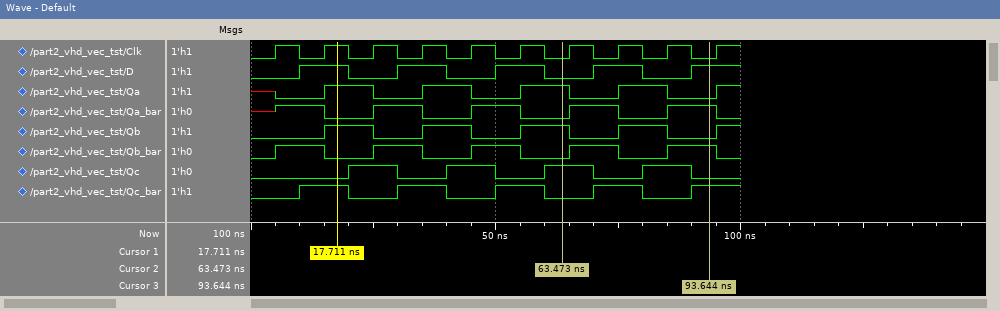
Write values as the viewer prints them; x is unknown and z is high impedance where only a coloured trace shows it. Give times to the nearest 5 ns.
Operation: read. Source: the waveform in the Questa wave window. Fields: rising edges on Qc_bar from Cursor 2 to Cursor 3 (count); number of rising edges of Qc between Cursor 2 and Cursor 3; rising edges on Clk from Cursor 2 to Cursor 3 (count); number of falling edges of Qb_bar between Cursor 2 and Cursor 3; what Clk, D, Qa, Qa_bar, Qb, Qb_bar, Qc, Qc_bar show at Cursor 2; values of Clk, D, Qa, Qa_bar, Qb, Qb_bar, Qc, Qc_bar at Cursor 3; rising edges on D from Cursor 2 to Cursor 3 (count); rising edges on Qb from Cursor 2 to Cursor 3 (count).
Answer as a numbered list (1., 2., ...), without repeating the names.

1. 2
2. 1
3. 3
4. 1
5. Clk=0, D=0, Qa=1, Qa_bar=0, Qb=1, Qb_bar=0, Qc=1, Qc_bar=0
6. Clk=0, D=1, Qa=0, Qa_bar=1, Qb=0, Qb_bar=1, Qc=0, Qc_bar=1
7. 2
8. 1
